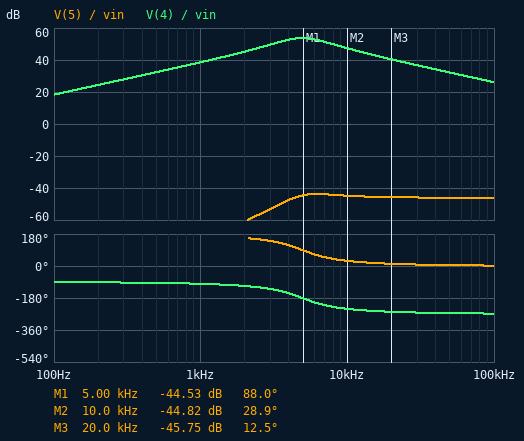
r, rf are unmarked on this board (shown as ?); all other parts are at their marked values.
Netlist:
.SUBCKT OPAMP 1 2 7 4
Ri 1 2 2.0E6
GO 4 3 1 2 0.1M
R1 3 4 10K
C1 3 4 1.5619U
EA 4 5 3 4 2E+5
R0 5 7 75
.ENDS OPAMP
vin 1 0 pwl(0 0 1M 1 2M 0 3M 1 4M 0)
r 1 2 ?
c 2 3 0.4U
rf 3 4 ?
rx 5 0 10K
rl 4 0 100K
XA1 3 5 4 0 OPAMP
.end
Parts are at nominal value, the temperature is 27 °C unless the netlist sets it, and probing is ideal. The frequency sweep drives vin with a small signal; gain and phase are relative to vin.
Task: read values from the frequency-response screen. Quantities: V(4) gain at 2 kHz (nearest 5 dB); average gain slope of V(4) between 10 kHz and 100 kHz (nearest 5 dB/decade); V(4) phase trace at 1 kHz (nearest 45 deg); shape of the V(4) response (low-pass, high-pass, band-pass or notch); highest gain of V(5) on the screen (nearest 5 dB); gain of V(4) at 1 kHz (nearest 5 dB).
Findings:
45 dB
-20 dB/decade
-90 deg
band-pass
-45 dB
40 dB
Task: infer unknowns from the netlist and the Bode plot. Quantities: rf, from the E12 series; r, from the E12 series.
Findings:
33 kΩ
68 Ω
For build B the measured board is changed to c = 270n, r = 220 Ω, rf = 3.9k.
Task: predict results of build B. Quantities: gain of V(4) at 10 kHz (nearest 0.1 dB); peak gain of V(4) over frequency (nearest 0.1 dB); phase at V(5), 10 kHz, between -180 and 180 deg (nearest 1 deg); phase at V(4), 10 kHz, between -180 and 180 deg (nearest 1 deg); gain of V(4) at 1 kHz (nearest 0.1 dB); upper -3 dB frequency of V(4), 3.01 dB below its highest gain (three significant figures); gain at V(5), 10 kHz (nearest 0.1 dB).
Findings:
24.8 dB
25.0 dB
100 deg
-170 deg
15.9 dB
109 kHz
-67.2 dB
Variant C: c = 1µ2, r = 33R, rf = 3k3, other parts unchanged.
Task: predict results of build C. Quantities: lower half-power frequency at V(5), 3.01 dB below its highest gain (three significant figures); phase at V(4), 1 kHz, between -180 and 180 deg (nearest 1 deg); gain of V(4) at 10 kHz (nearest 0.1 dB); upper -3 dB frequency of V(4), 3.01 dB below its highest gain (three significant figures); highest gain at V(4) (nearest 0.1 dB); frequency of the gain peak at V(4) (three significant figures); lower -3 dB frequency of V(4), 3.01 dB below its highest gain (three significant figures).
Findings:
15.9 kHz
-104 deg
39.9 dB
23.1 kHz
40.0 dB
8.88 kHz
3.42 kHz
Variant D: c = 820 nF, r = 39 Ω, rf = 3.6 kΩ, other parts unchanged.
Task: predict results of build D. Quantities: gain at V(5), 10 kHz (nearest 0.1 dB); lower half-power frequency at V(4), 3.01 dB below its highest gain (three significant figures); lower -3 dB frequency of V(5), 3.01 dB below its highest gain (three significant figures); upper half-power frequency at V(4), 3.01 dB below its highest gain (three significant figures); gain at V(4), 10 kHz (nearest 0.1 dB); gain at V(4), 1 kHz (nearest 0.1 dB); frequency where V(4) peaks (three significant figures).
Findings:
-52.7 dB
4.15 kHz
16.8 kHz
25.5 kHz
39.3 dB
25.3 dB
10.3 kHz
